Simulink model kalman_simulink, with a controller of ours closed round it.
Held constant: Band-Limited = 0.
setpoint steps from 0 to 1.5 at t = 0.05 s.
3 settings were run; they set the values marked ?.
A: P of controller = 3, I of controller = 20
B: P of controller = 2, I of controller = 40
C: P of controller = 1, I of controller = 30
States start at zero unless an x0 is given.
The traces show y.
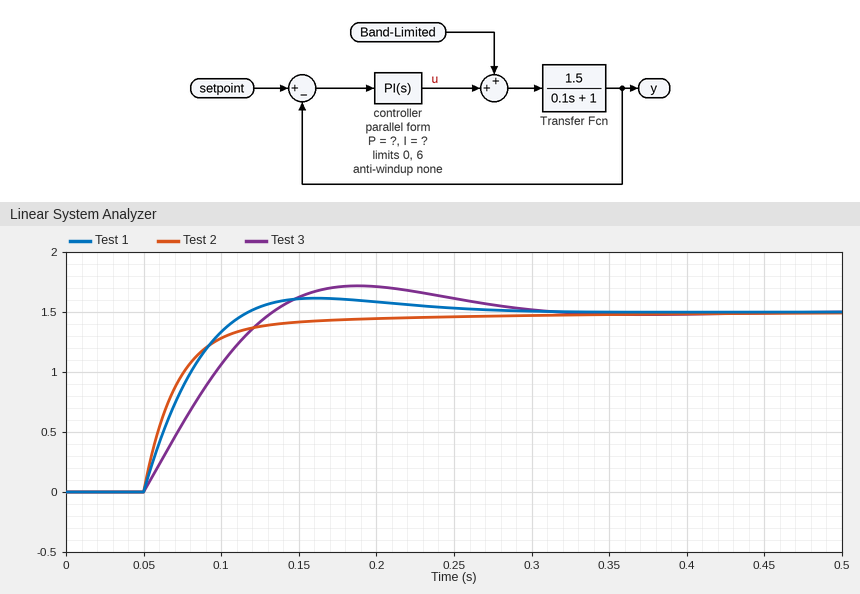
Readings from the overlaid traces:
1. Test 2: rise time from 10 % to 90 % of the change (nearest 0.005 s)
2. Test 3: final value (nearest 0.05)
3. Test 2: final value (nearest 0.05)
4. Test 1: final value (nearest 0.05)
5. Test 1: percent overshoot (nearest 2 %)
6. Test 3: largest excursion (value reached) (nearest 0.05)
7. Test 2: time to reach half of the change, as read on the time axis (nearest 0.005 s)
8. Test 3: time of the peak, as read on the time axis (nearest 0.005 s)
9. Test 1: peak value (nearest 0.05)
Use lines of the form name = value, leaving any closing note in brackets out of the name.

Test 2: rise time from 10 % to 90 % of the change = 0.060 s
Test 3: final value = 1.50
Test 2: final value = 1.50
Test 1: final value = 1.50
Test 1: percent overshoot = 8 %
Test 3: largest excursion (value reached) = 1.70
Test 2: time to reach half of the change, as read on the time axis = 0.065 s
Test 3: time of the peak, as read on the time axis = 0.190 s
Test 1: peak value = 1.60
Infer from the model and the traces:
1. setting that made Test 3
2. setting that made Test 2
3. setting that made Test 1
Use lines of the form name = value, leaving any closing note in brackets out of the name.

setting that made Test 3 = C
setting that made Test 2 = A
setting that made Test 1 = B
